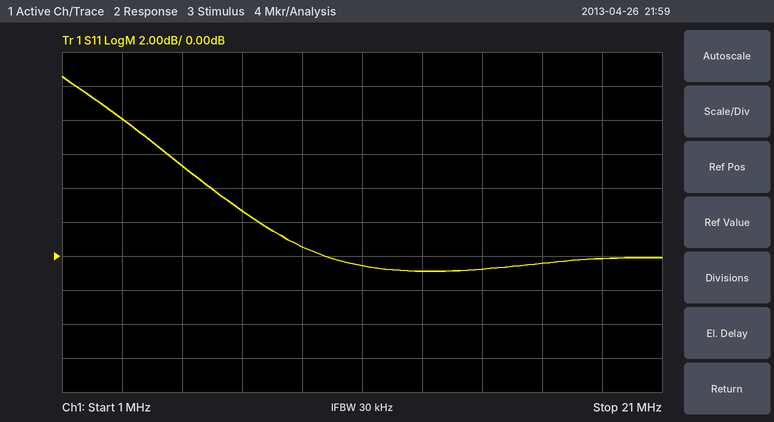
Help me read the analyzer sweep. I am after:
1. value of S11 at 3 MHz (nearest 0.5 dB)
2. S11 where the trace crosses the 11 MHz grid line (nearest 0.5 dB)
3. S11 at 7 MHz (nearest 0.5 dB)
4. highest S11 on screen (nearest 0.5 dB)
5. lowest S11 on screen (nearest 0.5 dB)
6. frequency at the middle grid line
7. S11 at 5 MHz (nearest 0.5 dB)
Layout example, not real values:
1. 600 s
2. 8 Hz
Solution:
1. 8.0 dB
2. -0.5 dB
3. 2.5 dB
4. 10.5 dB
5. -1.0 dB
6. 11 MHz
7. 5.5 dB
